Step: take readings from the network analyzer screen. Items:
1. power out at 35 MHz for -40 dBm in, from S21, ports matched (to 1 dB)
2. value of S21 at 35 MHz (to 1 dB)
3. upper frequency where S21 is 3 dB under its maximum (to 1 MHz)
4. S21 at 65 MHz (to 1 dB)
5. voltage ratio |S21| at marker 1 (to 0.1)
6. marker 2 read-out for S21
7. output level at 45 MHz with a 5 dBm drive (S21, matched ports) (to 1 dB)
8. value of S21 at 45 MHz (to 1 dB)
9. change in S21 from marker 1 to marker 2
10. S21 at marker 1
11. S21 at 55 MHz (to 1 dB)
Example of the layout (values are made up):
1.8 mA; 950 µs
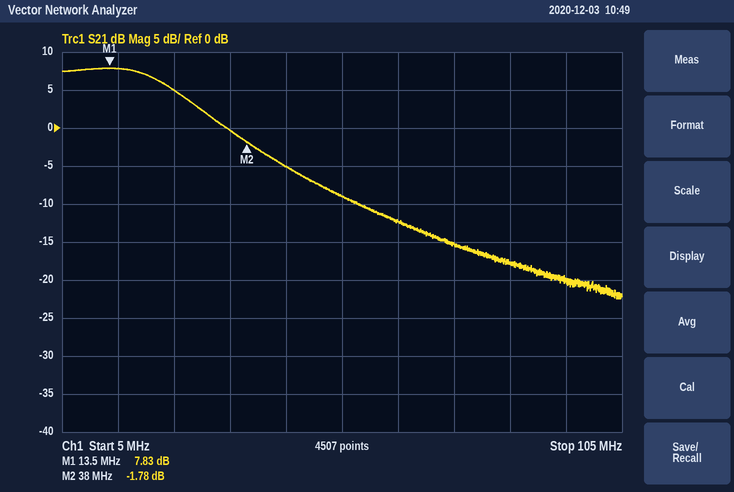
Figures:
-40 dBm; 0 dB; 25 MHz; -12 dB; 2.5; -1.78 dB; 0 dBm; -5 dB; -9.61 dB; 7.83 dB; -9 dB
